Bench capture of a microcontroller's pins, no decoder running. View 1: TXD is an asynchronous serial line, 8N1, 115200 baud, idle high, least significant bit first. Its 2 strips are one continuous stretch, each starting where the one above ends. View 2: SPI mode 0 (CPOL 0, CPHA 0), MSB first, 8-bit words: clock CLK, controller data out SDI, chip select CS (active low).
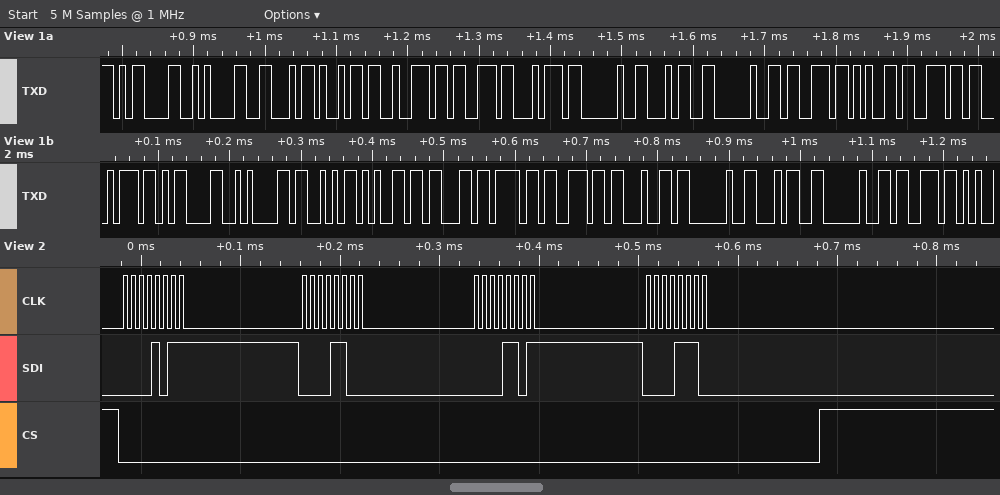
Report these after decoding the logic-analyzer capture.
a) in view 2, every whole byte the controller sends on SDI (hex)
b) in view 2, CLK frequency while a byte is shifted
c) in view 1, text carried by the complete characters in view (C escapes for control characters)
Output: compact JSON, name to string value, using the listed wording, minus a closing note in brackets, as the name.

{"in view 2, every whole byte the controller sends on SDI": "0B 0C 0D 0E", "in view 2, CLK frequency while a byte is shifted": "125 kHz", "in view 1, text carried by the complete characters in view": "\"\\r\\nFirst 4 sent\\r\\nSecond 4 s\""}
